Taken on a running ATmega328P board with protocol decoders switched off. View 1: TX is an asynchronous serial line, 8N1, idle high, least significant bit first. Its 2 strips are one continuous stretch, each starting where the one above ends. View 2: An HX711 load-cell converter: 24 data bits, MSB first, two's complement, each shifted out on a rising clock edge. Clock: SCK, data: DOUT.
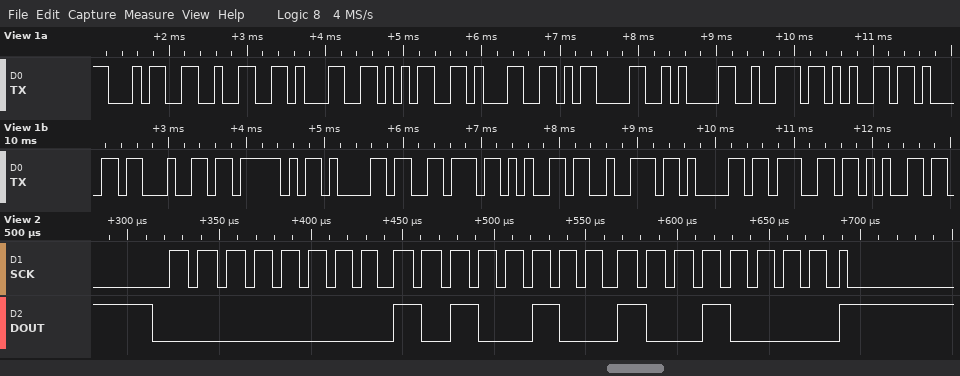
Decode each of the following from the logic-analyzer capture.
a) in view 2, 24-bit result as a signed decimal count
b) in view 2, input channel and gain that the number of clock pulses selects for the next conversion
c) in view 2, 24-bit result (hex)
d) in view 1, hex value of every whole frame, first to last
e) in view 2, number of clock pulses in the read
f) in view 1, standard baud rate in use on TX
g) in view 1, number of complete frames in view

42128
channel A, gain 128
0x00A490
0x34 0x32 0x31 0x35 0x31 0x0D 0x0A 0x72 0x65 0x61 0x64 0x5F 0x61 0x76 0x65 0x72 0x61 0x67 0x65
25
9600 baud
19
